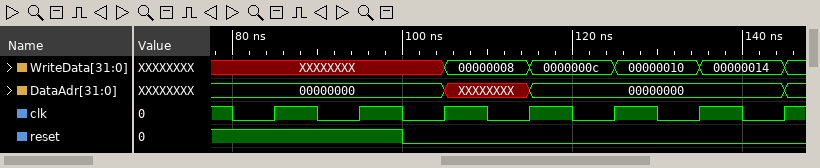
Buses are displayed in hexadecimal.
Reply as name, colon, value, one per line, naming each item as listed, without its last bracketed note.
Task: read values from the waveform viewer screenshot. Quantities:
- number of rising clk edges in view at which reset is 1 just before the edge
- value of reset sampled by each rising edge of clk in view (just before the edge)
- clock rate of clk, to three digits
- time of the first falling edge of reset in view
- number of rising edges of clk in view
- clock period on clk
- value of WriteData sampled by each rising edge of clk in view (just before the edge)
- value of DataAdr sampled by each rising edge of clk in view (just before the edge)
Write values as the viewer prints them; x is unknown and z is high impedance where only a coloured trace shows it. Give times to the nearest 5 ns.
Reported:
number of rising clk edges in view at which reset is 1 just before the edge: 2
value of reset sampled by each rising edge of clk in view: 1 1 0 0 0 0 0
clock rate of clk, to three digits: 100 MHz
time of the first falling edge of reset in view: 100 ns
number of rising edges of clk in view: 7
clock period on clk: 10 ns
value of WriteData sampled by each rising edge of clk in view: XXXXXXXX, XXXXXXXX, XXXXXXXX, 00000008, 0000000c, 00000010, 00000014
value of DataAdr sampled by each rising edge of clk in view: 00000000, 00000000, 00000000, XXXXXXXX, 00000000, 00000000, 00000000
